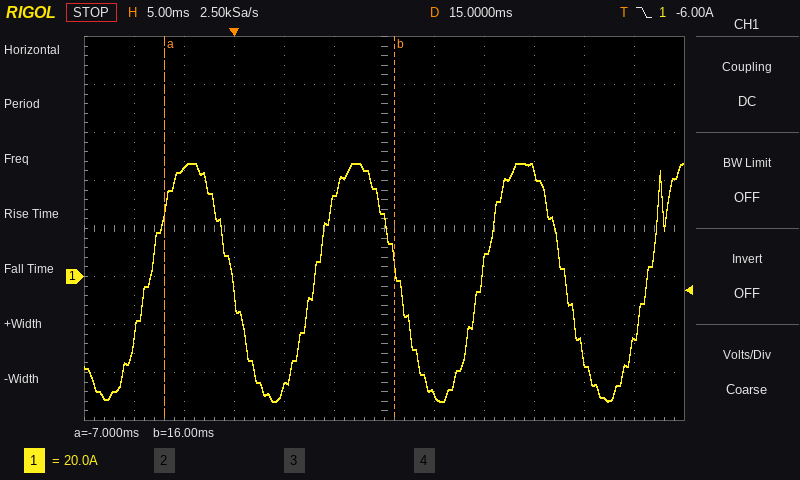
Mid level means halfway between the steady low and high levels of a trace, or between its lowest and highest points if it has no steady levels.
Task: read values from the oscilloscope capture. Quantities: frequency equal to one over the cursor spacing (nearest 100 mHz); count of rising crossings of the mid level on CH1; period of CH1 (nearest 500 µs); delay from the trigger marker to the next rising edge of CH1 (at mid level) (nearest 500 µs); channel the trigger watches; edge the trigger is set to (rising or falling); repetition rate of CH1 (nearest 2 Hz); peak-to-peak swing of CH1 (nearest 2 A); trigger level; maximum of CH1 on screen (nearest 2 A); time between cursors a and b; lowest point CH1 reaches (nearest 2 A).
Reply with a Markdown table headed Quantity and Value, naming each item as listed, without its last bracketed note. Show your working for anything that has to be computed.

| Quantity | Value |
|---|---|
| frequency equal to one over the cursor spacing | 1 / 23.0 ms ≈ 43.5 Hz |
| count of rising crossings of the mid level on CH1 | 4 |
| period of CH1 | 16.5 ms |
| delay from the trigger marker to the next rising edge of CH1 (at mid level) | 8.0 ms |
| channel the trigger watches | CH1 |
| edge the trigger is set to | falling |
| repetition rate of CH1 | 1 / 16.5 ms ≈ 60.6 Hz, so 60 Hz to the nearest 2 Hz |
| peak-to-peak swing of CH1 | 48 A − (-52 A) = 100 A |
| trigger level | -6.00 A |
| maximum of CH1 on screen | 48 A |
| time between cursors a and b | 16 ms − (-7 ms) = 23.0 ms |
| lowest point CH1 reaches | -52 A |
